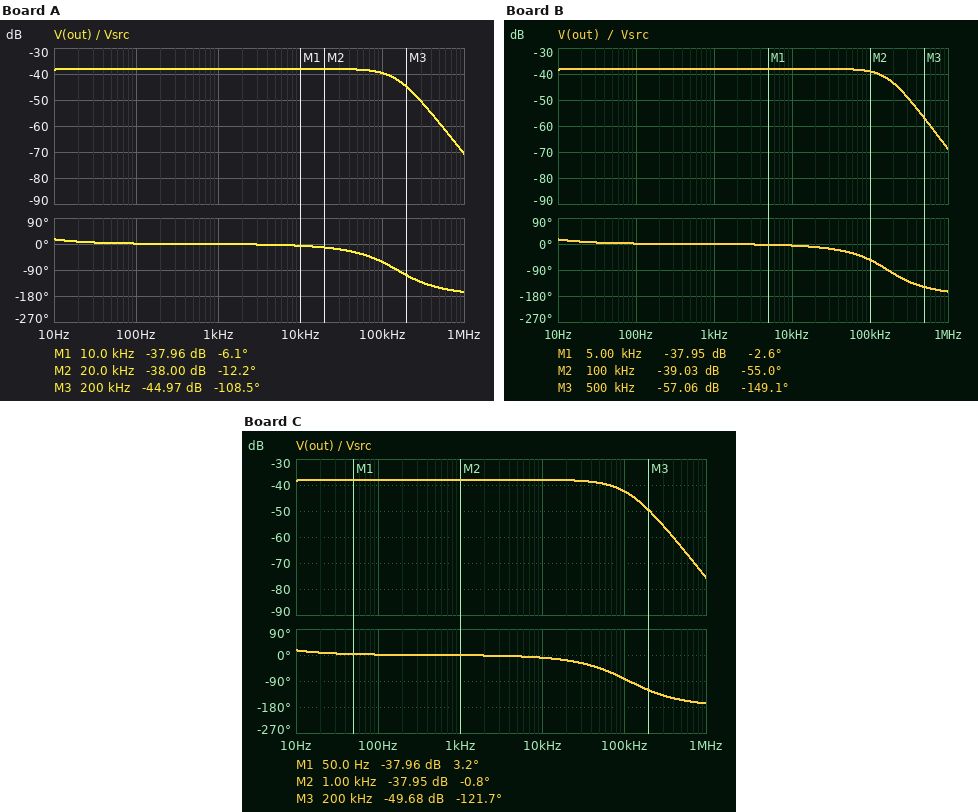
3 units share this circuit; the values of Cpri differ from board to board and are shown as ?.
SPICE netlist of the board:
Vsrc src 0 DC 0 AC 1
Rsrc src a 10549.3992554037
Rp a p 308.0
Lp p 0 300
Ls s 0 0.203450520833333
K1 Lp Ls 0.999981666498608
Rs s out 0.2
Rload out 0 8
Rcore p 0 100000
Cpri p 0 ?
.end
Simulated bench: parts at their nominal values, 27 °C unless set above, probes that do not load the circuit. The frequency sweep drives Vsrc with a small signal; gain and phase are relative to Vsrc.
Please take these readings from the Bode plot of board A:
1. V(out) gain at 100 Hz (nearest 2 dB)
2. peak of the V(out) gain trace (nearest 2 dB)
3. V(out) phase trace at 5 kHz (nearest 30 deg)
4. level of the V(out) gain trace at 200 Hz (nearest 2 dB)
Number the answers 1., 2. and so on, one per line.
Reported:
1. -38 dB
2. -38 dB
3. 0 deg
4. -38 dB
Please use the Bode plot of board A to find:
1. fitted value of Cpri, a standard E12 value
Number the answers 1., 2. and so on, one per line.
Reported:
1. 220 pF
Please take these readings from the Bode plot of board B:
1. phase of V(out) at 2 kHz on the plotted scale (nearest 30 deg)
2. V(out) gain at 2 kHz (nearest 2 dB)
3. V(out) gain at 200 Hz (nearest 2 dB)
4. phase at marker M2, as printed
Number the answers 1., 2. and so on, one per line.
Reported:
1. 0 deg
2. -38 dB
3. -38 dB
4. -55.0 deg
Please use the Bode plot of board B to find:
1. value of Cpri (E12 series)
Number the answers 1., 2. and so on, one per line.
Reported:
1. 180 pF
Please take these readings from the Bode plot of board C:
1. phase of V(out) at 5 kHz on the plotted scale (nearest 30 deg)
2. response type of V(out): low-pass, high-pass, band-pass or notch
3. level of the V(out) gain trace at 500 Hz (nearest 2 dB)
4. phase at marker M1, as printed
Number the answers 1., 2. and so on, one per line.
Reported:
1. 0 deg
2. low-pass
3. -38 dB
4. 3.2 deg
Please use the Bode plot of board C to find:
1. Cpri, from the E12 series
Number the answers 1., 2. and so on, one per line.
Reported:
1. 390 pF
